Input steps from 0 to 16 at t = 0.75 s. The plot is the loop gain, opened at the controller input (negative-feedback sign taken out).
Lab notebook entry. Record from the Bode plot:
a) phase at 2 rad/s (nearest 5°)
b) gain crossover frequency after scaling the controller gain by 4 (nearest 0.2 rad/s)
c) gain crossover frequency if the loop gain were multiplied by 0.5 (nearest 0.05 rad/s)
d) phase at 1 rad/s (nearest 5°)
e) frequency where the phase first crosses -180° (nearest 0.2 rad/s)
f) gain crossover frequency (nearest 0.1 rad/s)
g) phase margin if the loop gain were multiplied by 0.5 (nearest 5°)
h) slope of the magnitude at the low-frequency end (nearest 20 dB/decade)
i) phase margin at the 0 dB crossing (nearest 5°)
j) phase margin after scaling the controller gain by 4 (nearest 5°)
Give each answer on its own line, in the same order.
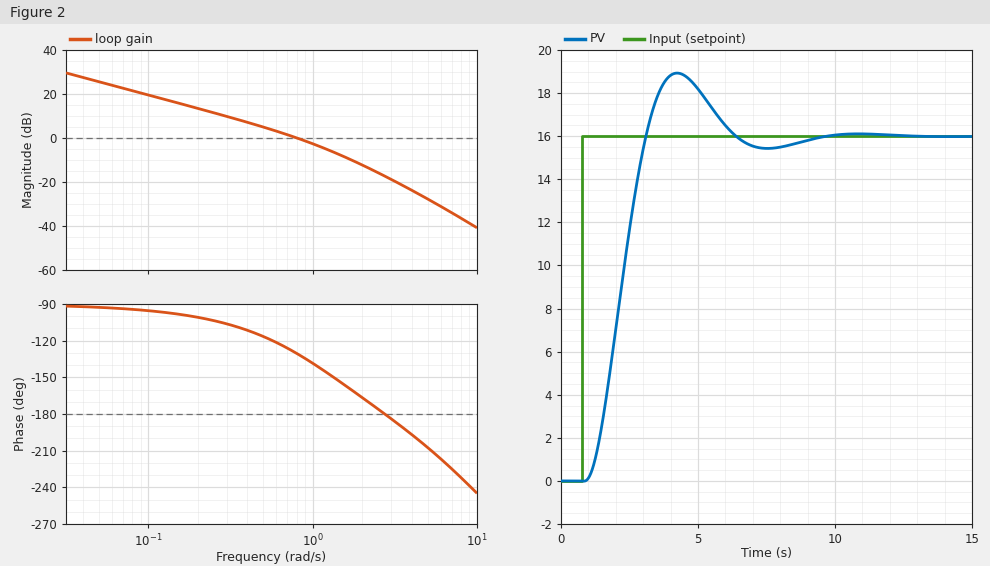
-165°
2.0 rad/s
0.45 rad/s
-140°
2.8 rad/s
0.8 rad/s
65°
-20 dB/decade
50°
15°
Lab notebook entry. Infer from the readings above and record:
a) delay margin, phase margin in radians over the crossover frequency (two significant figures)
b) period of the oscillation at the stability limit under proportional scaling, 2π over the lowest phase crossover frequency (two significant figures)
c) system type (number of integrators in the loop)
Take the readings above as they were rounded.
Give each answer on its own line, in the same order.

1.1 s
2.2 s
1
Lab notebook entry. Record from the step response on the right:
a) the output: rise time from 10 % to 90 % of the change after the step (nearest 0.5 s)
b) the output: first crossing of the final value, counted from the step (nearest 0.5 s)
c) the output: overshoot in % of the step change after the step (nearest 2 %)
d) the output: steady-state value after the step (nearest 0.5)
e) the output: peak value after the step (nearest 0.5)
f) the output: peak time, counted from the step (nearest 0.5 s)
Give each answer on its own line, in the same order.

1.5 s
2.5 s
18 %
16.0
19.0
3.5 s
